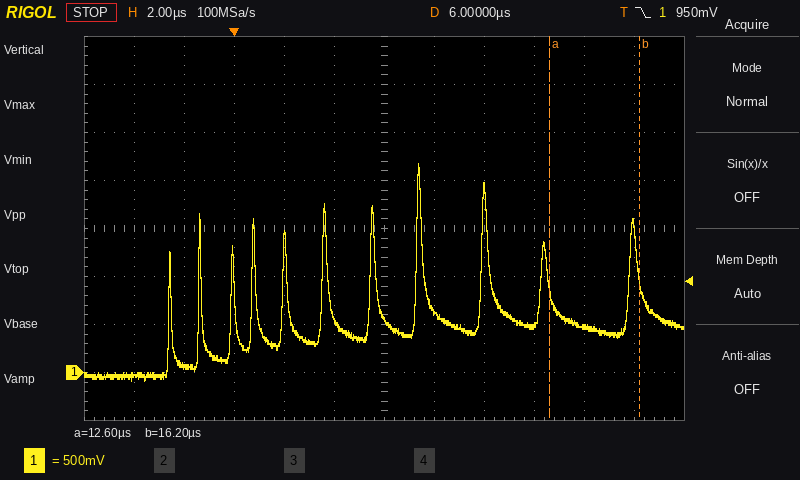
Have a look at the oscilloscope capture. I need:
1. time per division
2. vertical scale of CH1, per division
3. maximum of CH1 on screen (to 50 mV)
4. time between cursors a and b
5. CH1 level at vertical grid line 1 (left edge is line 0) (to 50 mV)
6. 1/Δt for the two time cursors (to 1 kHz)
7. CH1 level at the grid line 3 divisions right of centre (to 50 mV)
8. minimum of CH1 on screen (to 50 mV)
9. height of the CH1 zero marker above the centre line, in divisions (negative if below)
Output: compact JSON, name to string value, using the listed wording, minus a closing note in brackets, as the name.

{"time per division": "2 µs", "vertical scale of CH1, per division": "500 mV", "maximum of CH1 on screen": "2.20 V", "time between cursors a and b": "3.6 µs", "CH1 level at vertical grid line 1 (left edge is line 0)": "-50 mV", "1/Δt for the two time cursors": "278 kHz", "CH1 level at the grid line 3 divisions right of centre": "500 mV", "minimum of CH1 on screen": "-100 mV", "height of the CH1 zero marker above the centre line, in divisions": "-3.0 div"}
